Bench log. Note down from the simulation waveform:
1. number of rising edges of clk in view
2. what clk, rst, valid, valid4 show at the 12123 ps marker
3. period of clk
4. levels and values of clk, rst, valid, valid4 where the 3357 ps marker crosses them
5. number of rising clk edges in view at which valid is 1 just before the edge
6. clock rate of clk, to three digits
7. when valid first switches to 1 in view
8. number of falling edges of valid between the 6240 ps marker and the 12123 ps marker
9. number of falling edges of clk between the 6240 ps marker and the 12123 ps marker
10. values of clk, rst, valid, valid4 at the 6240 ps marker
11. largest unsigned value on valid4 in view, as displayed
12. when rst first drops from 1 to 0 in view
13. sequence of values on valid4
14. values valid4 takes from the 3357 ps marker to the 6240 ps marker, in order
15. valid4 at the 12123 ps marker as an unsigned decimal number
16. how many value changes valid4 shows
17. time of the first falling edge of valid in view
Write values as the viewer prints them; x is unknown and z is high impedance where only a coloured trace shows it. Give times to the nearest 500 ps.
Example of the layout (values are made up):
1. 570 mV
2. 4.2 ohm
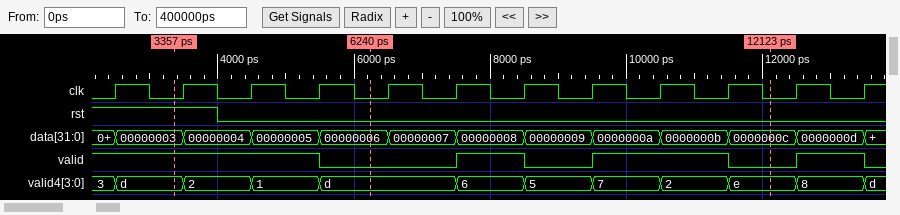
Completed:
1. 12
2. clk=0, rst=0, valid=0, valid4=e
3. 1000 ps
4. clk=0, rst=1, valid=1, valid4=d
5. 8
6. 1.00 GHz
7. 7500 ps
8. 2
9. 6
10. clk=0, rst=0, valid=0, valid4=d
11. e
12. 4000 ps
13. 3, d, 2, 1, d, 6, 5, 7, 2, e, 8, d
14. d, 2, 1, d
15. 14
16. 11
17. 5500 ps
